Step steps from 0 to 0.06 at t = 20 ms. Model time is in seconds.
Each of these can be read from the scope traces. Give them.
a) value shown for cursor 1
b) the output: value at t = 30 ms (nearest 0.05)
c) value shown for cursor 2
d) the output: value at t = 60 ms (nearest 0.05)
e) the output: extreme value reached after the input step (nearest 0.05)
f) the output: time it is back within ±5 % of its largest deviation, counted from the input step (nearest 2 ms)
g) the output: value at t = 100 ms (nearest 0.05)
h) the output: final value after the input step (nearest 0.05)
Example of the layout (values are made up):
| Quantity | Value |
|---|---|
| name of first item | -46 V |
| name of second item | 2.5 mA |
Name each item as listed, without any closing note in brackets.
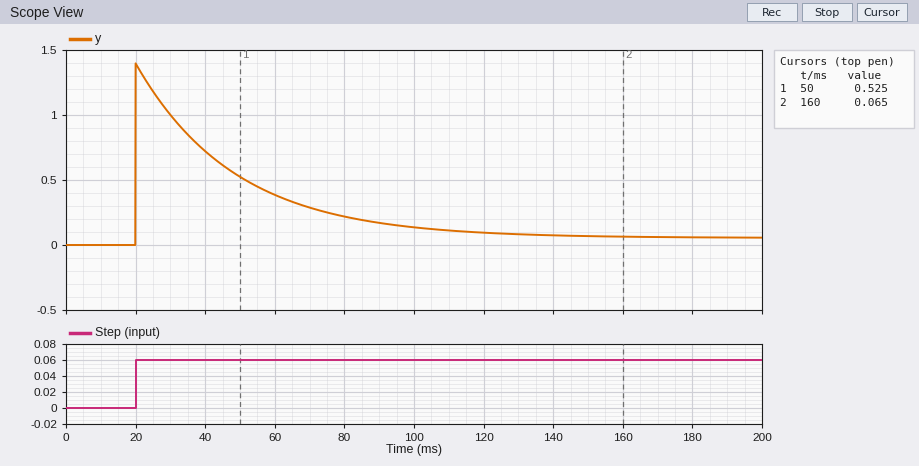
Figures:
| Quantity | Value |
|---|---|
| value shown for cursor 1 | 0.525 |
| the output: value at t = 30 ms | 1.00 |
| value shown for cursor 2 | 0.065 |
| the output: value at t = 60 ms | 0.40 |
| the output: extreme value reached after the input step | 1.40 |
| the output: time it is back within ±5 % of its largest deviation, counted from the input step | 84 ms |
| the output: value at t = 100 ms | 0.15 |
| the output: final value after the input step | 0.05 |
